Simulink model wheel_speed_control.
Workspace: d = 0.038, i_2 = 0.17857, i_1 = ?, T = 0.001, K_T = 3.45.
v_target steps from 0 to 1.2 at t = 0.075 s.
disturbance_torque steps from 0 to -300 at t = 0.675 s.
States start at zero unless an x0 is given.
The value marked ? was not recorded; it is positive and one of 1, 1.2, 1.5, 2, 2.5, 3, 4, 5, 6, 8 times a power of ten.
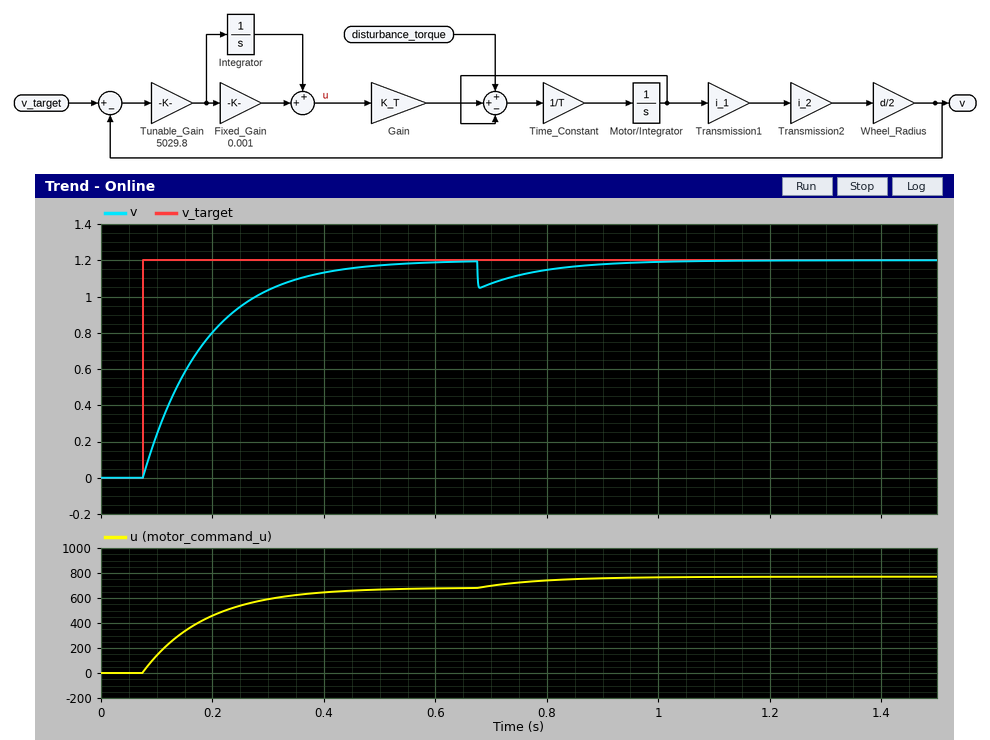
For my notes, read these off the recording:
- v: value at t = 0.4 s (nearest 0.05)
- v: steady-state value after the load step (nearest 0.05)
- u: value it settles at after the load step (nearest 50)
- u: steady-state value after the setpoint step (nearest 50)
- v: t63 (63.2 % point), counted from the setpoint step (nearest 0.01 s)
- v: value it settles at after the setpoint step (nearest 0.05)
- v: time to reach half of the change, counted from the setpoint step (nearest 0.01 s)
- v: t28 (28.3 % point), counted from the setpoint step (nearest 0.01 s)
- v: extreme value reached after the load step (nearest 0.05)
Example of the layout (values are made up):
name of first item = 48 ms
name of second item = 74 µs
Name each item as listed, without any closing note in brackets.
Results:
v: value at t = 0.4 s = 1.15
v: steady-state value after the load step = 1.20
u: value it settles at after the load step = 750
u: steady-state value after the setpoint step = 700
v: t63 (63.2 % point), counted from the setpoint step = 0.11 s
v: value it settles at after the setpoint step = 1.20
v: time to reach half of the change, counted from the setpoint step = 0.08 s
v: t28 (28.3 % point), counted from the setpoint step = 0.04 s
v: extreme value reached after the load step = 1.05
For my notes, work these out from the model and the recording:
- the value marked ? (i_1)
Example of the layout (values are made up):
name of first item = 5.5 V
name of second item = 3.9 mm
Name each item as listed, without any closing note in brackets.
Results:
the value marked ? = 0.15
